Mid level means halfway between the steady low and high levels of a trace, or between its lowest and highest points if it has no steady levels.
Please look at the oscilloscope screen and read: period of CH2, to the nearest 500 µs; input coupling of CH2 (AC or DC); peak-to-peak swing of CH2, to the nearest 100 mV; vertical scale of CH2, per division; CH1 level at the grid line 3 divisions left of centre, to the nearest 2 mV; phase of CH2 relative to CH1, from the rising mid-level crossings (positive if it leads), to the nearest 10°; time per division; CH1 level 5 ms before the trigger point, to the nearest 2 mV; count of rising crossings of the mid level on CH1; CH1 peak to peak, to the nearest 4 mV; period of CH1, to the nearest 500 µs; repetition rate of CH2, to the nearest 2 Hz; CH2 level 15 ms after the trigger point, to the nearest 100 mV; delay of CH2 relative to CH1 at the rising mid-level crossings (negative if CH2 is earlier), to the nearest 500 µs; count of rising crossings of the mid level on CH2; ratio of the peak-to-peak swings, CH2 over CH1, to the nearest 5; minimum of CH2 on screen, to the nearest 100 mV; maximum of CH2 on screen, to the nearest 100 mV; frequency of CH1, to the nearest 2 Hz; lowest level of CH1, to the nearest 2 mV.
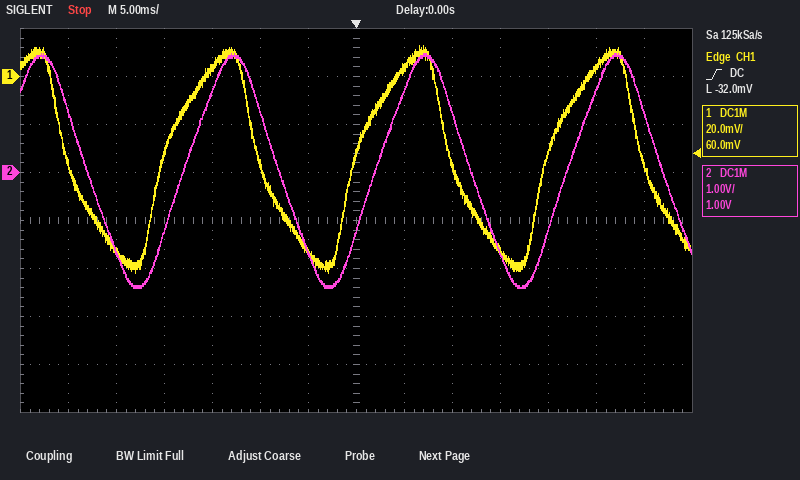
20.0 ms
DC
4.9 V
1 V
2 mV
-40°
5 ms
-72 mV
3
96 mV
20.0 ms
50 Hz
-1.7 V
+2.0 ms
3
50
-2.4 V
2.5 V
50 Hz
-82 mV
